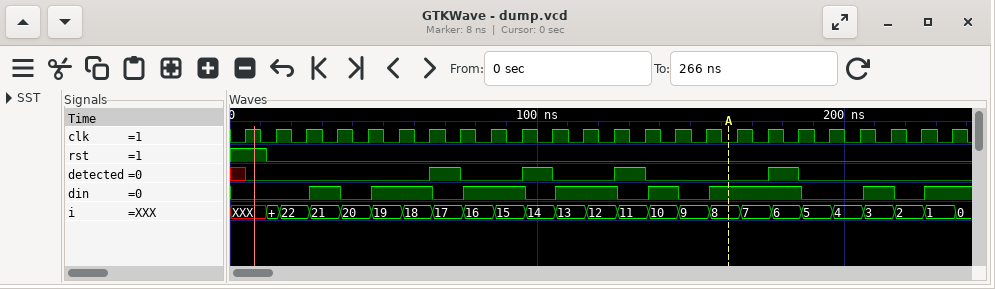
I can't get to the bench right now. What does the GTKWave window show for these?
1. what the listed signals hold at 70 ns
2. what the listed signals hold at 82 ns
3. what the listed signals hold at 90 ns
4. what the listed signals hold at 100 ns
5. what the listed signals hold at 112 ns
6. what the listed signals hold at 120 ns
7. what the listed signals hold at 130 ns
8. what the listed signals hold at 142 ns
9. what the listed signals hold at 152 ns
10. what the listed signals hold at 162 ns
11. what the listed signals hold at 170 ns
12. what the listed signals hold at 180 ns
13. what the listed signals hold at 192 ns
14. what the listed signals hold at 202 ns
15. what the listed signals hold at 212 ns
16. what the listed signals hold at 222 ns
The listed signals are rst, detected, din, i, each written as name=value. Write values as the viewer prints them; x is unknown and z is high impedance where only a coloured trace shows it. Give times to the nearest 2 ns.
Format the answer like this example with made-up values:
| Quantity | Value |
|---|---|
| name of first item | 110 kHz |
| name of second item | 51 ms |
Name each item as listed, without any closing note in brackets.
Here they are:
| Quantity | Value |
|---|---|
| what the listed signals hold at 70 ns | rst=0, detected=1, din=0, i=17 |
| what the listed signals hold at 82 ns | rst=0, detected=0, din=1, i=16 |
| what the listed signals hold at 90 ns | rst=0, detected=0, din=1, i=15 |
| what the listed signals hold at 100 ns | rst=0, detected=1, din=0, i=14 |
| what the listed signals hold at 112 ns | rst=0, detected=0, din=1, i=13 |
| what the listed signals hold at 120 ns | rst=0, detected=0, din=1, i=12 |
| what the listed signals hold at 130 ns | rst=0, detected=1, din=0, i=11 |
| what the listed signals hold at 142 ns | rst=0, detected=0, din=1, i=10 |
| what the listed signals hold at 152 ns | rst=0, detected=0, din=0, i=9 |
| what the listed signals hold at 162 ns | rst=0, detected=0, din=1, i=8 |
| what the listed signals hold at 170 ns | rst=0, detected=0, din=1, i=7 |
| what the listed signals hold at 180 ns | rst=0, detected=1, din=1, i=6 |
| what the listed signals hold at 192 ns | rst=0, detected=0, din=0, i=5 |
| what the listed signals hold at 202 ns | rst=0, detected=0, din=0, i=4 |
| what the listed signals hold at 212 ns | rst=0, detected=0, din=1, i=3 |
| what the listed signals hold at 222 ns | rst=0, detected=0, din=0, i=2 |
